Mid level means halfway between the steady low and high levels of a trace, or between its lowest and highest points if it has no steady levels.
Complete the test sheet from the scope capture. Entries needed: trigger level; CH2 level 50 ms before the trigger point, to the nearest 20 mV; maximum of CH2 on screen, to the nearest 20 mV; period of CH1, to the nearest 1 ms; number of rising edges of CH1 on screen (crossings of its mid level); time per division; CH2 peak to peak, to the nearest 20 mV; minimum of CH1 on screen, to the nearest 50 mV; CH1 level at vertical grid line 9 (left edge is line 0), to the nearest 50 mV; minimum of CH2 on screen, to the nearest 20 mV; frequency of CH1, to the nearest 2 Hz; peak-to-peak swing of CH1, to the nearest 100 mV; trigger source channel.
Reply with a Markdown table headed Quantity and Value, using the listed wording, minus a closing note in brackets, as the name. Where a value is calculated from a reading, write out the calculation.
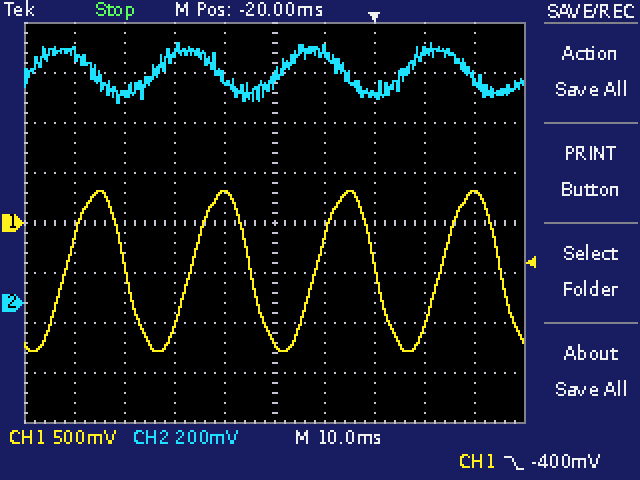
| Quantity | Value |
|---|---|
| trigger level | -400 mV |
| CH2 level 50 ms before the trigger point, to the nearest 20 mV | 840 mV |
| maximum of CH2 on screen, to the nearest 20 mV | 1.04 V |
| period of CH1, to the nearest 1 ms | 25 ms |
| number of rising edges of CH1 on screen | 4 |
| time per division | 10 ms |
| CH2 peak to peak, to the nearest 20 mV | 1.04 V − (800 mV) = 240 mV |
| minimum of CH1 on screen, to the nearest 50 mV | -1.30 V |
| CH1 level at vertical grid line 9 (left edge is line 0), to the nearest 50 mV | 300 mV |
| minimum of CH2 on screen, to the nearest 20 mV | 800 mV |
| frequency of CH1, to the nearest 2 Hz | 1 / 25 ms ≈ 40 Hz |
| peak-to-peak swing of CH1, to the nearest 100 mV | 1.60 V |
| trigger source channel | CH1 |
